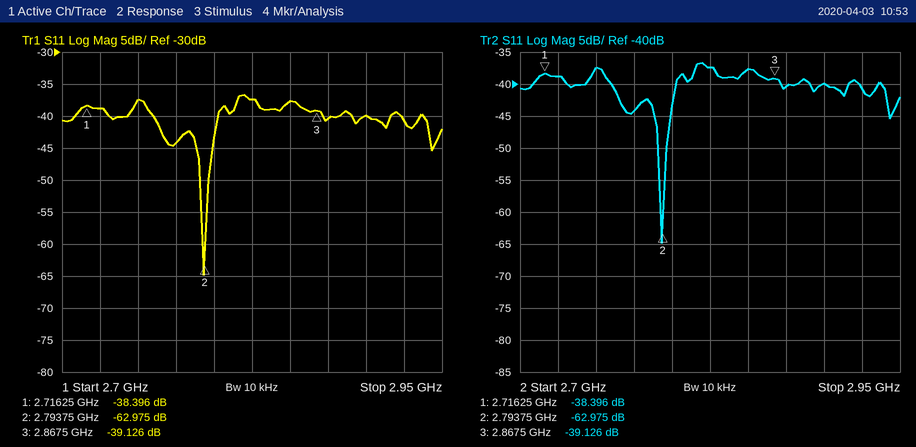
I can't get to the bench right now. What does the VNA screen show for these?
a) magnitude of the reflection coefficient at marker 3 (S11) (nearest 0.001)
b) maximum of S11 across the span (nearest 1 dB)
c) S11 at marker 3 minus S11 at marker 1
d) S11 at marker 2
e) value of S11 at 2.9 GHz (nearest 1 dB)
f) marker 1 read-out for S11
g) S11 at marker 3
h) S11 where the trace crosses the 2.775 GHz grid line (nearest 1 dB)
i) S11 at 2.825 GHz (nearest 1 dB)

0.011
-37 dB
-0.730 dB
-62.975 dB
-40 dB
-38.396 dB
-39.126 dB
-44 dB
-37 dB
